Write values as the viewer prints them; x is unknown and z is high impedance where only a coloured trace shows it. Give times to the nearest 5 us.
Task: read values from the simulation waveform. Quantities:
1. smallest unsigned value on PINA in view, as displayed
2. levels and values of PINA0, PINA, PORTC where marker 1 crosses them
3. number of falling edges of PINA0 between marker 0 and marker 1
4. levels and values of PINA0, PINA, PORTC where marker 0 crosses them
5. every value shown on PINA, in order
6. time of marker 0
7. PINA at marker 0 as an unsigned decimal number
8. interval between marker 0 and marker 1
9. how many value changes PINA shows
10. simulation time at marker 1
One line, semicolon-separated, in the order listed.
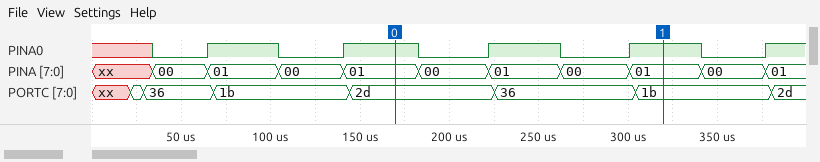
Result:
00; PINA0=1, PINA=01, PORTC=1b; 2; PINA0=1, PINA=01, PORTC=2d; xx, 00, 01, 00, 01, 00, 01, 00, 01, 00, 01; 170 us; 1; 150 us; 10; 320 us
